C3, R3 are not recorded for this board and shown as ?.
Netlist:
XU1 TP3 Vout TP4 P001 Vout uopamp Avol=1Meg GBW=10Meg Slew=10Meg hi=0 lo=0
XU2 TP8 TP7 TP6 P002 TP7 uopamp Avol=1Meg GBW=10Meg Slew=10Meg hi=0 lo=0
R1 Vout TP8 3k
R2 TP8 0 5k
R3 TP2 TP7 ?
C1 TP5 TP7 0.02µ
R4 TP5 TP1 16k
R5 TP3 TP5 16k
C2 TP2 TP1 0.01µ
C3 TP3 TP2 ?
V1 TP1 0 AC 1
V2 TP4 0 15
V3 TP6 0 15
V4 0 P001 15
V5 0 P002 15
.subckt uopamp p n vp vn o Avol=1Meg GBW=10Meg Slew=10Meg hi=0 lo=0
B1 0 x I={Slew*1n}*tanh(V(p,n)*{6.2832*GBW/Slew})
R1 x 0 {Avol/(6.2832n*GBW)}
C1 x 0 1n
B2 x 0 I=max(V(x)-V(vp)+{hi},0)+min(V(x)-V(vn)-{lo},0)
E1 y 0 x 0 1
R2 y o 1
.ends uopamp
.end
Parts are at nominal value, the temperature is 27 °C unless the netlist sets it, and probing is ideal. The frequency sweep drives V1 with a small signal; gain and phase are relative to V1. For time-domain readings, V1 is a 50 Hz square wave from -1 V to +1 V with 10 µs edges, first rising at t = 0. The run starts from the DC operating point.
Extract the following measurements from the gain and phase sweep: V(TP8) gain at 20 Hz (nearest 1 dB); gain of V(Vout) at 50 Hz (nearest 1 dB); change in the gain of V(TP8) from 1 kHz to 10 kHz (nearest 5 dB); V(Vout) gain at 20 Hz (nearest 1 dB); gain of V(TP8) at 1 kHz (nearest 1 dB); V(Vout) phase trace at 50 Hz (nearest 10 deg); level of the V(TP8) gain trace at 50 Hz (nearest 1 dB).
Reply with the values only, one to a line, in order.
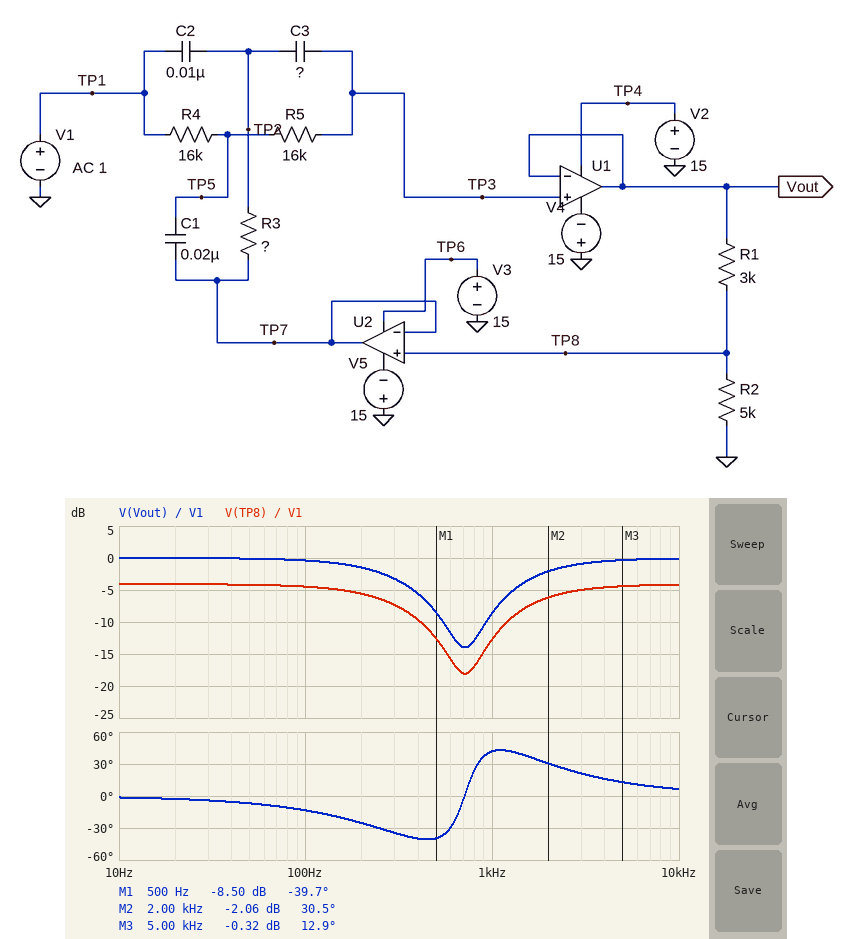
-4 dB
0 dB
10 dB
0 dB
-13 dB
-10 deg
-4 dB
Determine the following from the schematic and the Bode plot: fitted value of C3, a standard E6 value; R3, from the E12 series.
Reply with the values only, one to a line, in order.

22 nF
10 kΩ
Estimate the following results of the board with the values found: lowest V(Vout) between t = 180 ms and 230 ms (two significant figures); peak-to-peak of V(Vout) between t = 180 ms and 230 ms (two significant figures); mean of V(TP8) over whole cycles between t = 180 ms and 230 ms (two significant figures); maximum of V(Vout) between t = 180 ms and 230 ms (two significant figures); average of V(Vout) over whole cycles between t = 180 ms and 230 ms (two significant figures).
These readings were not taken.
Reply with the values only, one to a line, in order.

-1.0 V
2.0 V
110 mV
1.0 V
180 mV
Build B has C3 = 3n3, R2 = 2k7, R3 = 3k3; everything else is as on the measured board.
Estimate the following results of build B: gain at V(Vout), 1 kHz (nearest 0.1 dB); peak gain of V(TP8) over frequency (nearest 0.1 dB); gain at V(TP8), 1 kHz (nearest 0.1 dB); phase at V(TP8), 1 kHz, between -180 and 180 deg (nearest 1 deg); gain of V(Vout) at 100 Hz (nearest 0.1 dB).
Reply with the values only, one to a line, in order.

-5.0 dB
-6.5 dB
-11.5 dB
-73 deg
-0.1 dB
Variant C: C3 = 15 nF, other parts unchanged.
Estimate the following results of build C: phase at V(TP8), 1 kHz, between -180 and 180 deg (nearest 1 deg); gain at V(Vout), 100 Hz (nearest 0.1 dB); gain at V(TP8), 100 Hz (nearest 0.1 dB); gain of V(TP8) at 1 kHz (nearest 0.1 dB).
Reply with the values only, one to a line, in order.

46 deg
-0.2 dB
-4.3 dB
-15.5 dB
